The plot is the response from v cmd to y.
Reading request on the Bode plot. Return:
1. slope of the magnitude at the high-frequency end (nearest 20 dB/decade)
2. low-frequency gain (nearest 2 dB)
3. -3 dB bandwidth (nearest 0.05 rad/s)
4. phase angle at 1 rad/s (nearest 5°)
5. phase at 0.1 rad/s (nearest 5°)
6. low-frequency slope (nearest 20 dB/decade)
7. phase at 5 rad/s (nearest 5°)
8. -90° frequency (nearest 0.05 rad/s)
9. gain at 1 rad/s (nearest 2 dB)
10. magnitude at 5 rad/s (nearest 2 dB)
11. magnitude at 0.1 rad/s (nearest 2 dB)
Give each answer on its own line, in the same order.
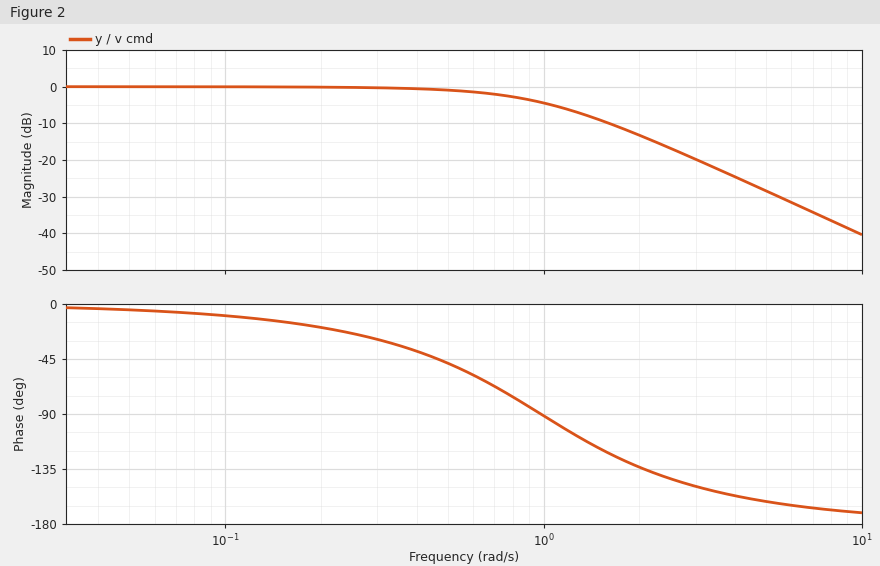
-40 dB/decade
0 dB
0.85 rad/s
-90°
-10°
0 dB/decade
-160°
1.00 rad/s
-4 dB
-28 dB
0 dB
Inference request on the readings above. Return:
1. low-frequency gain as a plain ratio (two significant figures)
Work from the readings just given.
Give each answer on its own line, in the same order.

1.0
